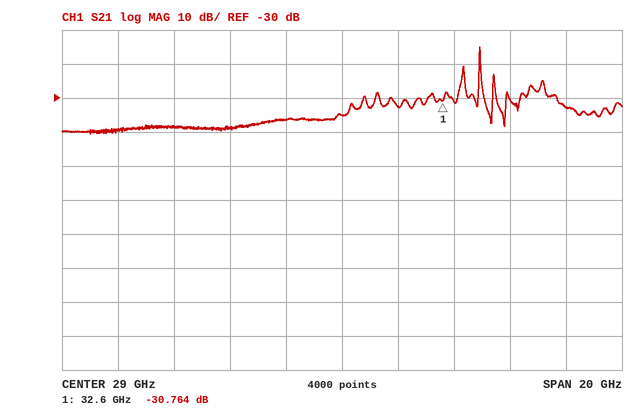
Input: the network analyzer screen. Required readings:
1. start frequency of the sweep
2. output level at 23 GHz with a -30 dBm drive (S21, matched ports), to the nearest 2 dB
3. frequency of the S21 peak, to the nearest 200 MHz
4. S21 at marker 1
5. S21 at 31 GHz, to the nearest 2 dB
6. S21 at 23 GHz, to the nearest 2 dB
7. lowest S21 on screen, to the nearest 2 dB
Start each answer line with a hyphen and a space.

- 19 GHz
- -68 dBm
- 34.0 GHz
- -30.764 dB
- -32 dB
- -38 dB
- -40 dB
